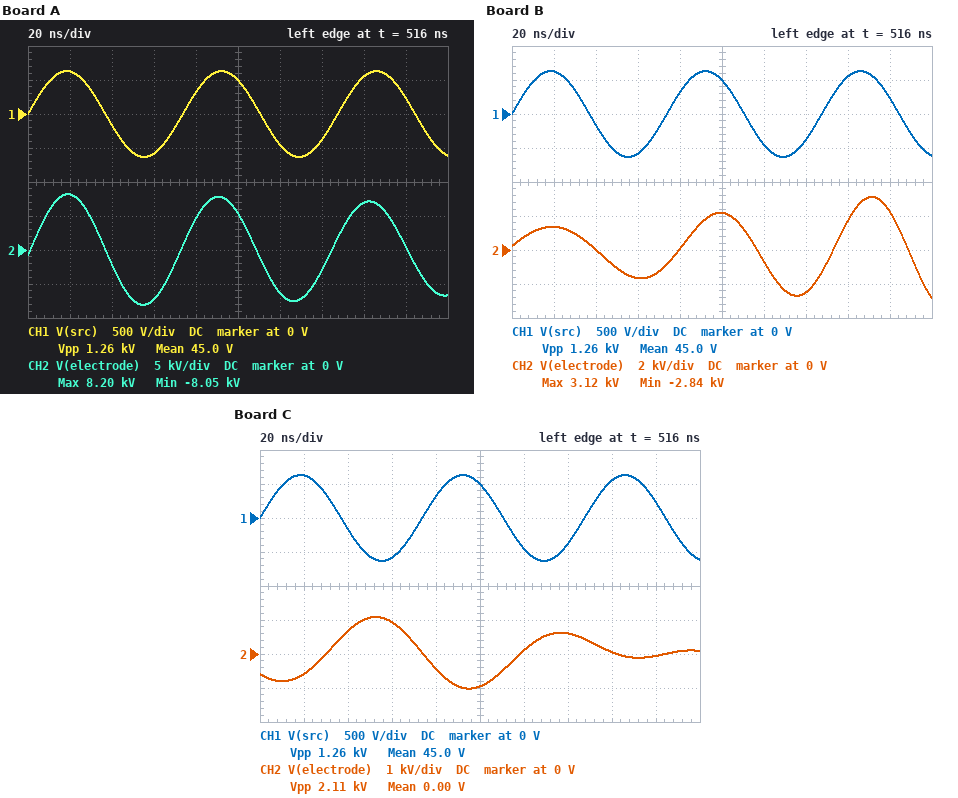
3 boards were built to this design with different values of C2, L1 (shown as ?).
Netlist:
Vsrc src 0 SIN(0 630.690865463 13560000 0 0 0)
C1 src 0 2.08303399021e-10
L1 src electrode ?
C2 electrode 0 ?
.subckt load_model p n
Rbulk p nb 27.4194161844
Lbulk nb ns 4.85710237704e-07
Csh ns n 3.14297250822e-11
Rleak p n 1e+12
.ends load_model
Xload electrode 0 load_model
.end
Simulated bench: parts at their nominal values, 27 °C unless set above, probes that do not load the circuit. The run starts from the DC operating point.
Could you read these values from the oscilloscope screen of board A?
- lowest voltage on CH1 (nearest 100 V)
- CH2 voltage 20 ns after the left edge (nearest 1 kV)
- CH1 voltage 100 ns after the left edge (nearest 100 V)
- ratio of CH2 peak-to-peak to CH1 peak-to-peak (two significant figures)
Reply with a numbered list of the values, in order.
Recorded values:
1. -600 V
2. 8 kV
3. 500 V
4. 13
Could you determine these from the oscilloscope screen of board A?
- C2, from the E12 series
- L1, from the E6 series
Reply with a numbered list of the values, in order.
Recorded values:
1. 220 pF
2. 470 nH
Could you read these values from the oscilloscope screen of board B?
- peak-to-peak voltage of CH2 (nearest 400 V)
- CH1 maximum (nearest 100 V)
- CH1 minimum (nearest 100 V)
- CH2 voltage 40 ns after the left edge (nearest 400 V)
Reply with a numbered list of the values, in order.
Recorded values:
1. 6.0 kV
2. 600 V
3. -600 V
4. 0 V
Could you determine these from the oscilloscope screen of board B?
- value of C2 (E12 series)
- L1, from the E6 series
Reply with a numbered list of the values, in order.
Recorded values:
1. 120 pF
2. 680 nH
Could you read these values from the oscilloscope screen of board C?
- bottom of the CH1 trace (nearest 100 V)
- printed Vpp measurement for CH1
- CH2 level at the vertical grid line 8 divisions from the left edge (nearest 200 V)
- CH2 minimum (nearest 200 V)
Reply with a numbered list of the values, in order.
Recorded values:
1. -600 V
2. 1.26 kV
3. 0 V
4. -1.0 kV
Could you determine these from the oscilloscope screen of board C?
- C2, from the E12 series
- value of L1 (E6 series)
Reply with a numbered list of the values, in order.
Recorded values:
1. 56 pF
2. 3.3 µH
